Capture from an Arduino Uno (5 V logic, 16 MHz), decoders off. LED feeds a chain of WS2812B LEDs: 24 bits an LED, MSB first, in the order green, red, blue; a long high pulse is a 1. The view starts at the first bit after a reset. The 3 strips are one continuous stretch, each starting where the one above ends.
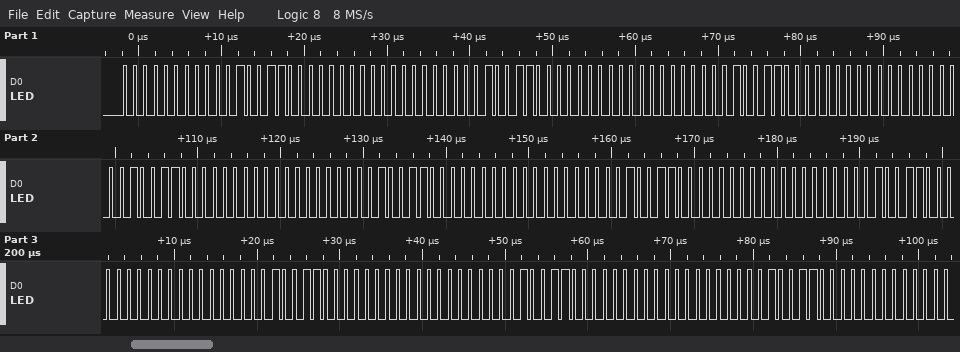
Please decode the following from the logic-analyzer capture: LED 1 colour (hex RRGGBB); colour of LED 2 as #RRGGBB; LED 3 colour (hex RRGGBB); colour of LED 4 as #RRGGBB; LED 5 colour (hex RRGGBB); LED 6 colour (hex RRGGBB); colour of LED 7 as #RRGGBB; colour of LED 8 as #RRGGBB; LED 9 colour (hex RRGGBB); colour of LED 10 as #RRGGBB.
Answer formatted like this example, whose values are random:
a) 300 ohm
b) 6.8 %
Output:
a) #130000
b) #130000
c) #130000
d) #130000
e) #130000
f) #130000
g) #130000
h) #130000
i) #130000
j) #130000
